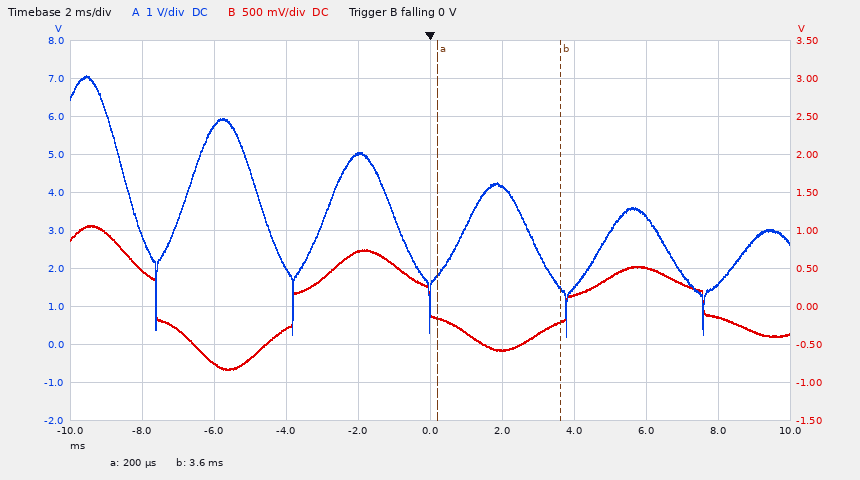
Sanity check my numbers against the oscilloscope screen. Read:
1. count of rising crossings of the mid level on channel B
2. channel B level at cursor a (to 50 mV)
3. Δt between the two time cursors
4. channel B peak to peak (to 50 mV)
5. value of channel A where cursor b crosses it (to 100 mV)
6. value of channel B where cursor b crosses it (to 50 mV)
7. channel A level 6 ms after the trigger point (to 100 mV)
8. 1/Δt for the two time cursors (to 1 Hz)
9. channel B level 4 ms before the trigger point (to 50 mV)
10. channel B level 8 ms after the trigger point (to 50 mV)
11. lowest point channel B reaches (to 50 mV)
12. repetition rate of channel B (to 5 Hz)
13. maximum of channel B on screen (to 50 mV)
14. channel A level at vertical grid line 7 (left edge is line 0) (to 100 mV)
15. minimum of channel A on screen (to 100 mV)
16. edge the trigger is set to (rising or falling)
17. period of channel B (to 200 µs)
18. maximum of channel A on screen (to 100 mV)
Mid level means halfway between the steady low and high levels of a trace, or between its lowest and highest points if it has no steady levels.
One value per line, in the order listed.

2
-150 mV
3.4 ms
1.90 V
1.5 V
-200 mV
3.4 V
294 Hz
-300 mV
-150 mV
-850 mV
130 Hz
1.05 V
1.5 V
200 mV
falling
7.6 ms
7.1 V
